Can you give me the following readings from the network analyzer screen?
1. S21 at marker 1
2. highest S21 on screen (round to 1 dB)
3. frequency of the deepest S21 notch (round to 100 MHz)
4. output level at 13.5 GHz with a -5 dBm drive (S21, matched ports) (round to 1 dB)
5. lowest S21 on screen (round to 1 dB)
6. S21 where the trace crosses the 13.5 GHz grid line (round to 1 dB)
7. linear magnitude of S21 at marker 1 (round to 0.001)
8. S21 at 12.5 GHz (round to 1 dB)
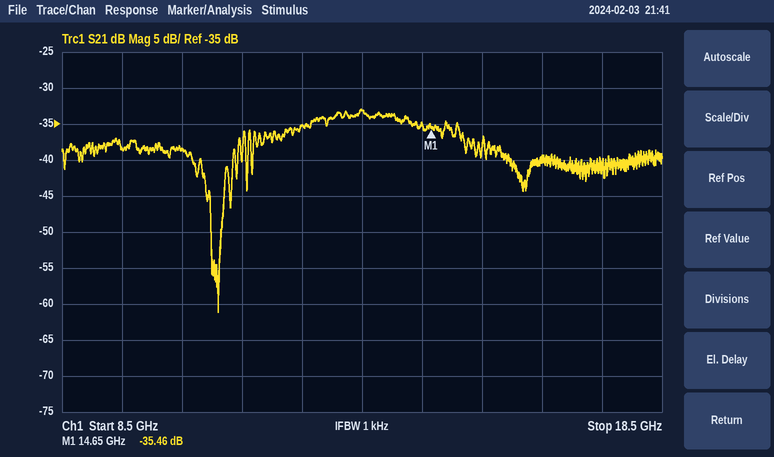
-35.46 dB
-33 dB
11.1 GHz
-38 dBm
-61 dB
-33 dB
0.017
-35 dB
